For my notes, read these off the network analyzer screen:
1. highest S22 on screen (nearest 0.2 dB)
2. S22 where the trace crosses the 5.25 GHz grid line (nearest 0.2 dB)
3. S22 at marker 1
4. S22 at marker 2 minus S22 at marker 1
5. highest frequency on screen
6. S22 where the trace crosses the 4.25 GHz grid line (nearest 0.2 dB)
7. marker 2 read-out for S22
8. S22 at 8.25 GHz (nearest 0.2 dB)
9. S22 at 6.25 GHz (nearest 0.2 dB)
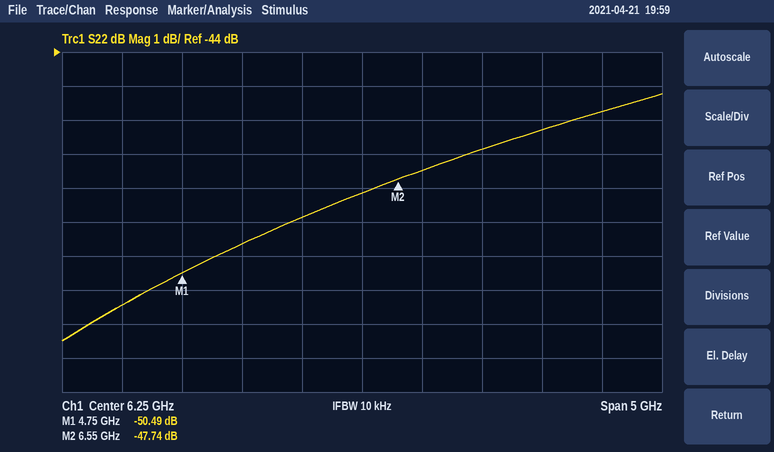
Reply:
-45.2 dB
-49.6 dB
-50.49 dB
2.75 dB
8.75 GHz
-51.4 dB
-47.74 dB
-45.8 dB
-48.2 dB
